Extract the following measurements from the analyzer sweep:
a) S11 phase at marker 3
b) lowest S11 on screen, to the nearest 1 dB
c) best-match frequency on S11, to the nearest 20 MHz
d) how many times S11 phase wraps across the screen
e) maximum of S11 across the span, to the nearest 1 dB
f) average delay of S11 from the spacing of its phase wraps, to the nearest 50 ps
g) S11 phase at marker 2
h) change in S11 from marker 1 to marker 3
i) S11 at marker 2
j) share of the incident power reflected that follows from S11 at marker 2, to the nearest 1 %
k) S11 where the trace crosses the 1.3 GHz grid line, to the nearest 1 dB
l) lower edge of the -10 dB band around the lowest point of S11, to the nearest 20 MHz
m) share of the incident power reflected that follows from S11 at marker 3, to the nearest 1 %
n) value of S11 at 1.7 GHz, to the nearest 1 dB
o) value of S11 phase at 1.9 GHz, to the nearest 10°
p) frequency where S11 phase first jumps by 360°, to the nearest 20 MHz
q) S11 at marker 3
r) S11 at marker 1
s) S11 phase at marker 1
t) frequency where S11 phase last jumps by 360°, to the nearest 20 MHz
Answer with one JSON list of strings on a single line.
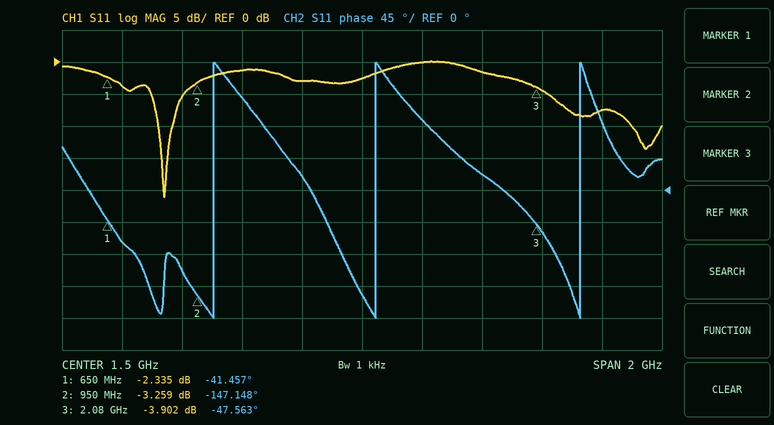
["-47.563°", "-21 dB", "840 MHz", "3", "0 dB", "1.65 ns", "-147.148°", "-1.567 dB", "-3.259 dB", "47 %", "-3 dB", "820 MHz", "41 %", "0 dB", "20°", "1.00 GHz", "-3.902 dB", "-2.335 dB", "-41.457°", "2.22 GHz"]
